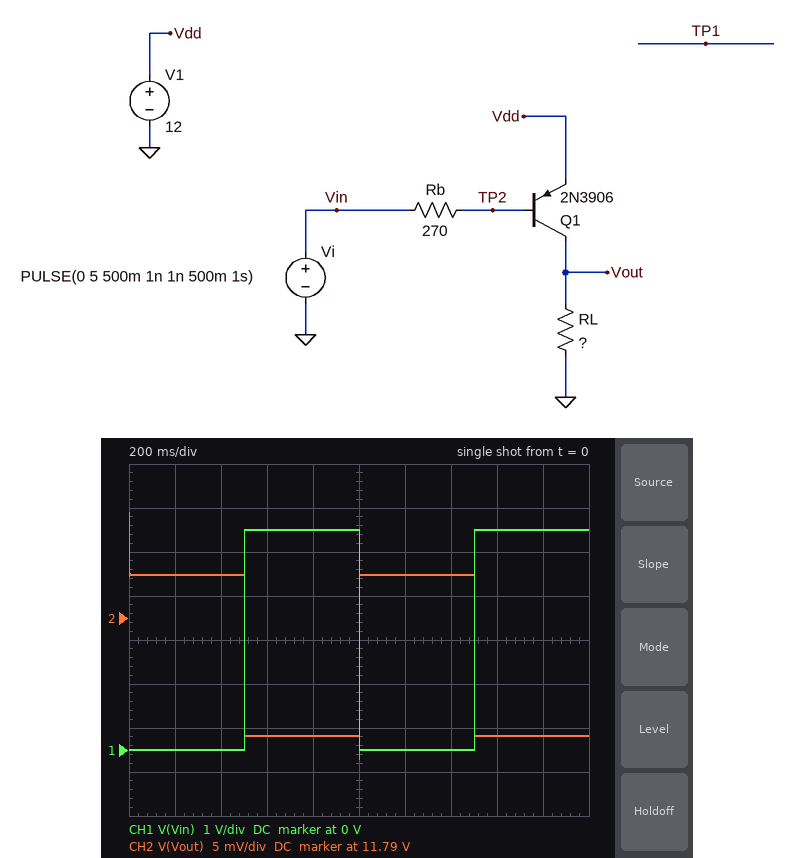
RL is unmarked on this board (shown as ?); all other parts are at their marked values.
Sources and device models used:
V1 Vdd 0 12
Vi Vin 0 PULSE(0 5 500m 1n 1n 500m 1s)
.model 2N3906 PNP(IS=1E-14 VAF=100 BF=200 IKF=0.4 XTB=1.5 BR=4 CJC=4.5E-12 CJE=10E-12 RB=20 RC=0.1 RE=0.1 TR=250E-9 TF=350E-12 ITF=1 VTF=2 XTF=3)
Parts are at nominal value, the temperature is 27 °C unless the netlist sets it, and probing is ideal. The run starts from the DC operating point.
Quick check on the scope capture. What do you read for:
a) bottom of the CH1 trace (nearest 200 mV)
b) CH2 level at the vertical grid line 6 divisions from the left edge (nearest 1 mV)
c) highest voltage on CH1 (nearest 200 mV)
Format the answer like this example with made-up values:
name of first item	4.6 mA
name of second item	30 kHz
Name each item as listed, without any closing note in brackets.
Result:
bottom of the CH1 trace	0 V
CH2 level at the vertical grid line 6 divisions from the left edge	11.790 V
highest voltage on CH1	5.0 V
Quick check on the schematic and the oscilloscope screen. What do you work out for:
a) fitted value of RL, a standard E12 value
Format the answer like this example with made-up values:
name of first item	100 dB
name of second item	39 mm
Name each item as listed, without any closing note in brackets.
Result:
fitted value of RL, a standard E12 value	18 Ω
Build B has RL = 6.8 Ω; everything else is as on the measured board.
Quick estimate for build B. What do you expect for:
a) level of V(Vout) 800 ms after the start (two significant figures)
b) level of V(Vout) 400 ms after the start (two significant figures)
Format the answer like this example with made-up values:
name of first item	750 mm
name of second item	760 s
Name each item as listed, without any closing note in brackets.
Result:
level of V(Vout) 800 ms after the start	7.7 V
level of V(Vout) 400 ms after the start	11 V
